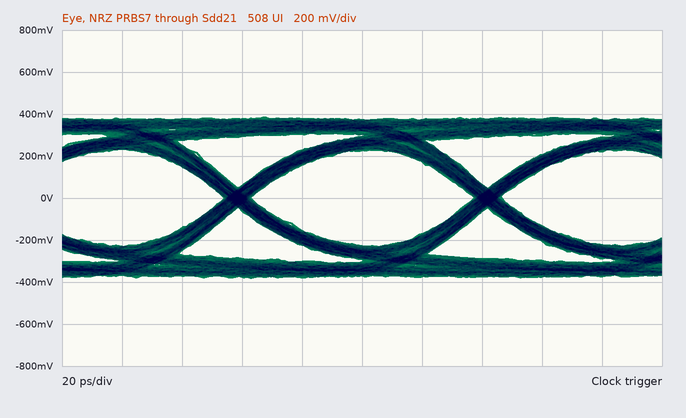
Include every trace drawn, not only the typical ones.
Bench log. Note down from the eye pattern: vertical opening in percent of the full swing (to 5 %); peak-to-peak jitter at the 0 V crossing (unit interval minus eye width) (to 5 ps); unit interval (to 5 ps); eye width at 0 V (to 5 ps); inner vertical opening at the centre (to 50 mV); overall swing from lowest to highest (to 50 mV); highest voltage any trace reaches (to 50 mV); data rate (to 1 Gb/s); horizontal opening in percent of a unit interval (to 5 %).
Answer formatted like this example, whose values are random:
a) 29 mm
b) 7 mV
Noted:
a) 60 %
b) 10 ps
c) 85 ps
d) 75 ps
e) 450 mV
f) 750 mV
g) 400 mV
h) 12 Gb/s
i) 90 %
